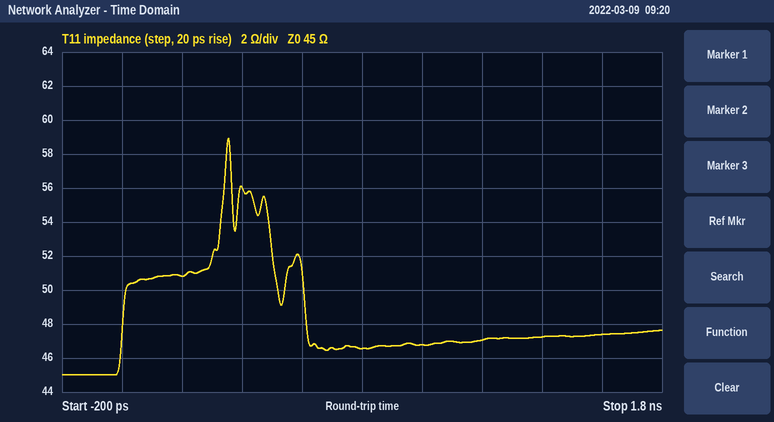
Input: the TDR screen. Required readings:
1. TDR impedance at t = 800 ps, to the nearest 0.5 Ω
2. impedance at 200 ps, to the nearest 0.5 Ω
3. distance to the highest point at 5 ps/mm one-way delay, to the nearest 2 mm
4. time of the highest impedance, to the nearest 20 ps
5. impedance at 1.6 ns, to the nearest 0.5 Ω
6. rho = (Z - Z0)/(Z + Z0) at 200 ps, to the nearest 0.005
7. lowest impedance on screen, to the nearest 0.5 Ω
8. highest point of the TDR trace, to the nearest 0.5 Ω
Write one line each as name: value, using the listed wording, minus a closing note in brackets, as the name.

TDR impedance at t = 800 ps, to the nearest 0.5 Ω: 46.5 Ω
impedance at 200 ps, to the nearest 0.5 Ω: 51.0 Ω
distance to the highest point at 5 ps/mm one-way delay, to the nearest 2 mm: 36 mm
time of the highest impedance, to the nearest 20 ps: 360 ps
impedance at 1.6 ns, to the nearest 0.5 Ω: 47.5 Ω
rho = (Z - Z0)/(Z + Z0) at 200 ps, to the nearest 0.005: +0.060
lowest impedance on screen, to the nearest 0.5 Ω: 45.0 Ω
highest point of the TDR trace, to the nearest 0.5 Ω: 59.0 Ω
